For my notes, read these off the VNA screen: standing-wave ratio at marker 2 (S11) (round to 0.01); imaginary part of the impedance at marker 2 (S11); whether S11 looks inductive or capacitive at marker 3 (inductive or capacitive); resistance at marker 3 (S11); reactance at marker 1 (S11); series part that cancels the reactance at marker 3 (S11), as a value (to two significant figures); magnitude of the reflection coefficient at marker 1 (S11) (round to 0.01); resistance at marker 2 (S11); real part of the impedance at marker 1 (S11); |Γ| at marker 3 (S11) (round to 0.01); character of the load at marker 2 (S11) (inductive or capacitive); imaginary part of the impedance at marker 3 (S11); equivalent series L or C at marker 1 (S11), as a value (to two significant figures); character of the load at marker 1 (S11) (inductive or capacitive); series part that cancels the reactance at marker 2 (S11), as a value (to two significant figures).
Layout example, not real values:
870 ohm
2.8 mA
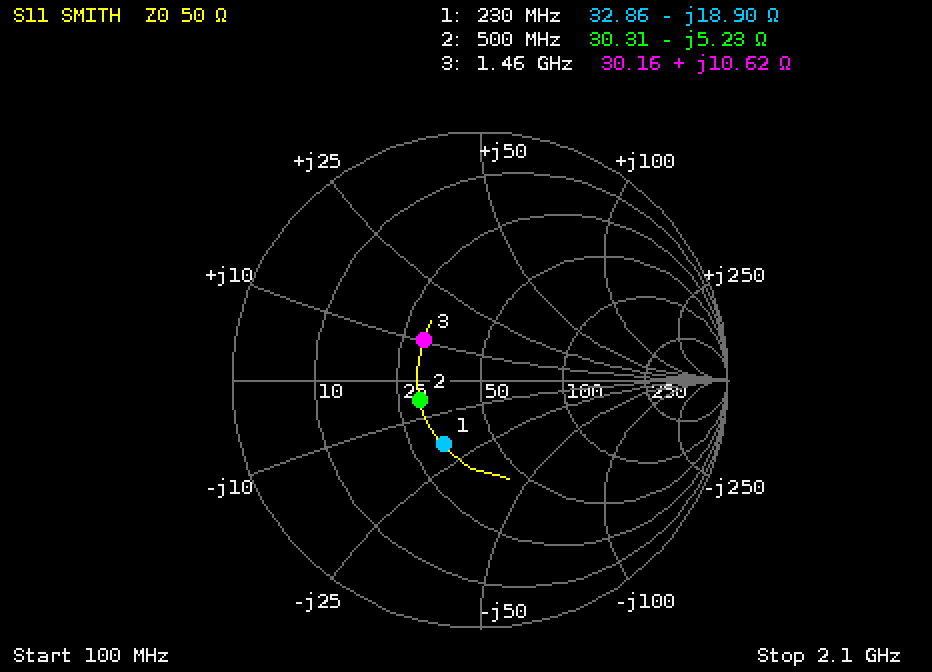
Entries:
1.68
-5.23 Ω
inductive
30.16 Ω
-18.90 Ω
10 pF
0.30
30.31 Ω
32.86 Ω
0.28
capacitive
+10.62 Ω
37 pF
capacitive
1.7 nH
